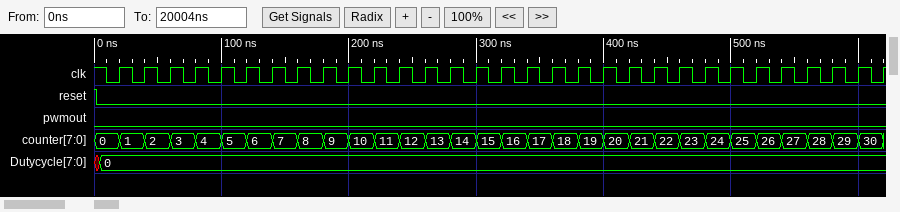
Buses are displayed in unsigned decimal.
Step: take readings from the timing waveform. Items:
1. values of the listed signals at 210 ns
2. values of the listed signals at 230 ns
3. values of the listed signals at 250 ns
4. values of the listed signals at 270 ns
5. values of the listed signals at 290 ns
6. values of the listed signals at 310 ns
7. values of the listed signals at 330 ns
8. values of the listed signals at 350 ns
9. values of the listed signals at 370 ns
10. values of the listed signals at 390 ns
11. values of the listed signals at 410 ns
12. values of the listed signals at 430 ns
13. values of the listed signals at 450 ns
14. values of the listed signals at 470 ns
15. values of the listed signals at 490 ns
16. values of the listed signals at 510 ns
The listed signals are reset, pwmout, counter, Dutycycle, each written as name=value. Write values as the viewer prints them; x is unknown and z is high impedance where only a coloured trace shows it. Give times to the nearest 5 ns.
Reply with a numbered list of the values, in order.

1. reset=0, pwmout=0, counter=10, Dutycycle=0
2. reset=0, pwmout=0, counter=11, Dutycycle=0
3. reset=0, pwmout=0, counter=12, Dutycycle=0
4. reset=0, pwmout=0, counter=13, Dutycycle=0
5. reset=0, pwmout=0, counter=14, Dutycycle=0
6. reset=0, pwmout=0, counter=15, Dutycycle=0
7. reset=0, pwmout=0, counter=16, Dutycycle=0
8. reset=0, pwmout=0, counter=17, Dutycycle=0
9. reset=0, pwmout=0, counter=18, Dutycycle=0
10. reset=0, pwmout=0, counter=19, Dutycycle=0
11. reset=0, pwmout=0, counter=20, Dutycycle=0
12. reset=0, pwmout=0, counter=21, Dutycycle=0
13. reset=0, pwmout=0, counter=22, Dutycycle=0
14. reset=0, pwmout=0, counter=23, Dutycycle=0
15. reset=0, pwmout=0, counter=24, Dutycycle=0
16. reset=0, pwmout=0, counter=25, Dutycycle=0
